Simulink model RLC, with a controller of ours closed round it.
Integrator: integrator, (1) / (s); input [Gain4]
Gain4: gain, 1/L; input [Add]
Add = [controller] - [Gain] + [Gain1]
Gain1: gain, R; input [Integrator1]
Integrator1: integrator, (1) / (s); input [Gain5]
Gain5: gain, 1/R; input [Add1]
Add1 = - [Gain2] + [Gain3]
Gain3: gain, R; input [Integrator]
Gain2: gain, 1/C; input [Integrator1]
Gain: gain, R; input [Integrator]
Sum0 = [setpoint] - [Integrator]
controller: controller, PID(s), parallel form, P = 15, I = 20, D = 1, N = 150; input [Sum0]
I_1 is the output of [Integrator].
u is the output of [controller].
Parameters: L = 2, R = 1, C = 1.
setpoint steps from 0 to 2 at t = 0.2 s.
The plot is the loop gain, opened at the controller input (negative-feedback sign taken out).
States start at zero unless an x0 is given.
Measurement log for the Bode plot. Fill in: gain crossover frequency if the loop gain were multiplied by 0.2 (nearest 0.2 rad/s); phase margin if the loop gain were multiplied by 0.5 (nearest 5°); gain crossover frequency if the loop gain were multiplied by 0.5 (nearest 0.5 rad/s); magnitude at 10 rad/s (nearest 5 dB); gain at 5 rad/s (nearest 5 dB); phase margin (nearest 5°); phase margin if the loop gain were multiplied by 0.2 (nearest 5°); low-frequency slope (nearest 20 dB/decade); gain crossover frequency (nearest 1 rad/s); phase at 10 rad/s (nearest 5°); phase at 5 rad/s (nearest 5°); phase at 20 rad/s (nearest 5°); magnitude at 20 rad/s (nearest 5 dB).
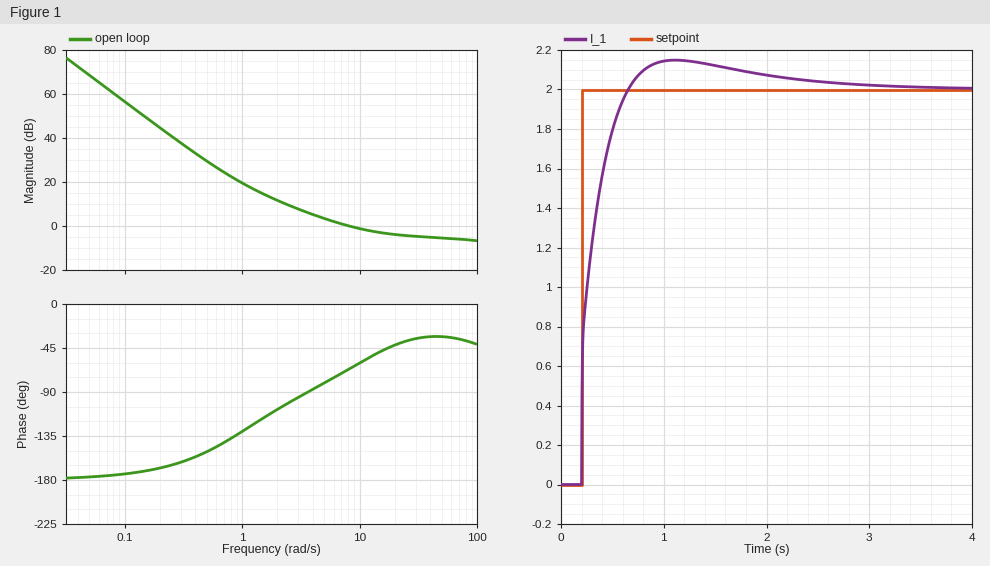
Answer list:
1.6 rad/s
90°
3.5 rad/s
0 dB
5 dB
115°
65°
-40 dB/decade
8 rad/s
-60°
-80°
-40°
-5 dB
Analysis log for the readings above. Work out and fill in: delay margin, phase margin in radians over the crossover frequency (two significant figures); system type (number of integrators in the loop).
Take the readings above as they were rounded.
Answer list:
0.25 s
2
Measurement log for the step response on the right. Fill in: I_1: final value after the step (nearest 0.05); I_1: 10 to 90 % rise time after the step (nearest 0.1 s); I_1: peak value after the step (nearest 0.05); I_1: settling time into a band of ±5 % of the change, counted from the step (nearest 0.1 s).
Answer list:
2.00
0.3 s
2.15
1.5 s
